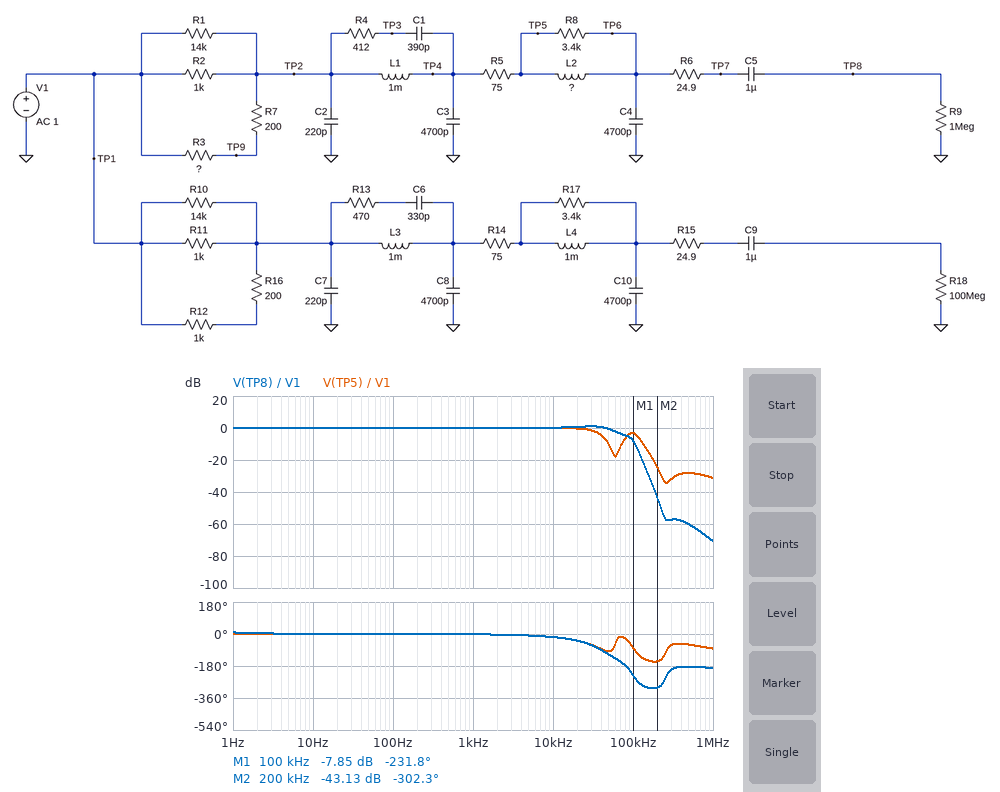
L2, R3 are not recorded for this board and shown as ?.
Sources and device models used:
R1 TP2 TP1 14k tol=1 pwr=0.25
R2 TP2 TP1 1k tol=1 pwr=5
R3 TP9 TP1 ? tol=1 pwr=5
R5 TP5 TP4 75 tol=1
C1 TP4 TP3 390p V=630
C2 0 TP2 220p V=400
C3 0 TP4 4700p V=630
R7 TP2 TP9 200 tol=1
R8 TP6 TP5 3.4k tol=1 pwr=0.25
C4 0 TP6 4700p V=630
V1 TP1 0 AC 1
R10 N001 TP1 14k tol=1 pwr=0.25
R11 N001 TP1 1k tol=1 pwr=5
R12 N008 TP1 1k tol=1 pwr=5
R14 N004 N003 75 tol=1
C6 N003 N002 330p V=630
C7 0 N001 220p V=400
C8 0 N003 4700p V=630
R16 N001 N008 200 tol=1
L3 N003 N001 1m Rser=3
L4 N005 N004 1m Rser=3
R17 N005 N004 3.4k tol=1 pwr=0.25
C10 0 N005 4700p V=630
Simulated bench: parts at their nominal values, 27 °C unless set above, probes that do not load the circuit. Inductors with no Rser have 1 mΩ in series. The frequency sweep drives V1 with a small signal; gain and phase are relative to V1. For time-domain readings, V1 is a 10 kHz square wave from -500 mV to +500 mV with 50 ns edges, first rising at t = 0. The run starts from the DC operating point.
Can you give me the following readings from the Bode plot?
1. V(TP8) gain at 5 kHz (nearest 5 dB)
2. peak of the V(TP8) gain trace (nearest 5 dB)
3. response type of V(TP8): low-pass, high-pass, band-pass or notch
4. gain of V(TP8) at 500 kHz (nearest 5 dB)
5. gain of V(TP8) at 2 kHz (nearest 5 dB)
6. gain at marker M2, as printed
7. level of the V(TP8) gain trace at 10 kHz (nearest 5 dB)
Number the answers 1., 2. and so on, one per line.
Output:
1. 0 dB
2. 0 dB
3. low-pass
4. -60 dB
5. 0 dB
6. -43.13 dB
7. 0 dB
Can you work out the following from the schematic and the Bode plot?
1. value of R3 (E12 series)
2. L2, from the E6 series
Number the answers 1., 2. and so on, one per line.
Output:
1. 680 Ω
2. 1.5 mH
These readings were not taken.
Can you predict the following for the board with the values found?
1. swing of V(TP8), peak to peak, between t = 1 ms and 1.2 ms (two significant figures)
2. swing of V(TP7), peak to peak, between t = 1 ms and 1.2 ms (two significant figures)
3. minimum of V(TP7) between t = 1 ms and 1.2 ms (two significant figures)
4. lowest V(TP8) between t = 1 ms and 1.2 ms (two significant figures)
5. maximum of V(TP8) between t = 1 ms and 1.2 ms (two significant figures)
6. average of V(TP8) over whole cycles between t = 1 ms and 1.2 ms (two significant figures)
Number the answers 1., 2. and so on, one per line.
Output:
1. 1.3 V
2. 1.3 V
3. -640 mV
4. -140 mV
5. 1.1 V
6. 500 mV
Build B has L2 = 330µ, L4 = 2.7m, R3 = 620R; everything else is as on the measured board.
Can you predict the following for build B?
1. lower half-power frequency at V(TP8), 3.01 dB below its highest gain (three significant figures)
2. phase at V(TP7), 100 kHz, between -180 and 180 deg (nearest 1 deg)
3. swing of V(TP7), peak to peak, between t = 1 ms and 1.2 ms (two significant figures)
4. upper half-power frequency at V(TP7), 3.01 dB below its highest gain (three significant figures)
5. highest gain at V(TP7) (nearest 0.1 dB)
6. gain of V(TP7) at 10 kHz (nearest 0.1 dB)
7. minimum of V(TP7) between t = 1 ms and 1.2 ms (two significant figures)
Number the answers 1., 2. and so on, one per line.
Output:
1. 162 mHz
2. -155 deg
3. 1.1 V
4. 55.8 kHz
5. 0.1 dB
6. 0 dB
7. -560 mV
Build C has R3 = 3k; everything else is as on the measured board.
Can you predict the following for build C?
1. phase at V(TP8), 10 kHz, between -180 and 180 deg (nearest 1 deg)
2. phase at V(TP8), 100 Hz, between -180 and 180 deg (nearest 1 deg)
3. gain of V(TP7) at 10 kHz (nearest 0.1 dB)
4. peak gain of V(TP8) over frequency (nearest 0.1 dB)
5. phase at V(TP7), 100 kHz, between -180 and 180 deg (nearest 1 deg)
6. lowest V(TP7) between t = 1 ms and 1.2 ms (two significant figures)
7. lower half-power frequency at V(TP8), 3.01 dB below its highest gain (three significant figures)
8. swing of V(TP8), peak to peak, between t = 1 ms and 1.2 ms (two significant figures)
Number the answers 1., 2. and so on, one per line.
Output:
1. -26 deg
2. 0 deg
3. -0.3 dB
4. 0 dB
5. 133 deg
6. -500 mV
7. 159 mHz
8. 1.0 V
